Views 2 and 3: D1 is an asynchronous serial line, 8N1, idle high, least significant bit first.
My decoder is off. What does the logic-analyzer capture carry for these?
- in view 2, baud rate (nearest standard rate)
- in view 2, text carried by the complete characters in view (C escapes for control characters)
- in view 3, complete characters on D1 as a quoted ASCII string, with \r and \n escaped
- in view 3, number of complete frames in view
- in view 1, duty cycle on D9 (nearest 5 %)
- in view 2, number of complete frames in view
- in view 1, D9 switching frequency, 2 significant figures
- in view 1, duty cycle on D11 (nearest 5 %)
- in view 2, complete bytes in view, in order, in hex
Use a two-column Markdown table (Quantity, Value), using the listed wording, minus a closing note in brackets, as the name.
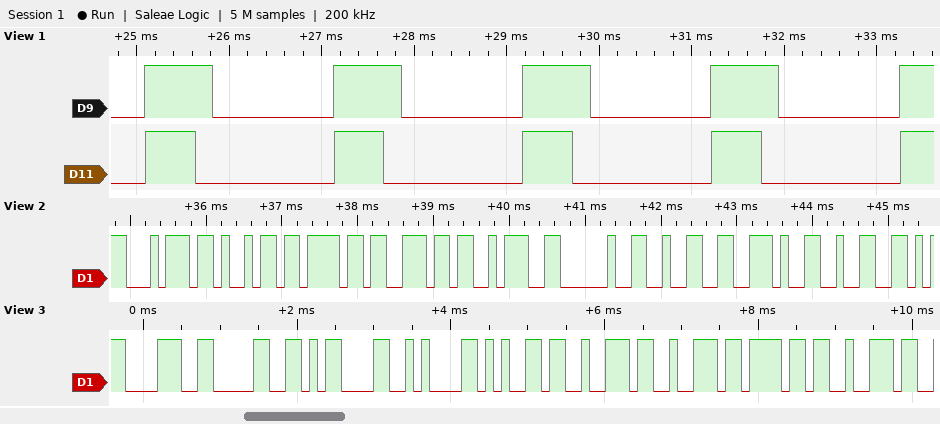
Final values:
| Quantity | Value |
|---|---|
| in view 2, baud rate | 9600 baud |
| in view 2, text carried by the complete characters in view | "tion: 2.2" |
| in view 3, complete characters on D1 as a quoted ASCII string, with \r and \n escaped | "80\r\nerror" |
| in view 3, number of complete frames in view | 9 |
| in view 1, duty cycle on D9 | 35 % |
| in view 2, number of complete frames in view | 9 |
| in view 1, D9 switching frequency, 2 significant figures | 490 Hz |
| in view 1, duty cycle on D11 | 25 % |
| in view 2, complete bytes in view, in order, in hex | 74 69 6F 6E 3A 20 32 2E 32 |
